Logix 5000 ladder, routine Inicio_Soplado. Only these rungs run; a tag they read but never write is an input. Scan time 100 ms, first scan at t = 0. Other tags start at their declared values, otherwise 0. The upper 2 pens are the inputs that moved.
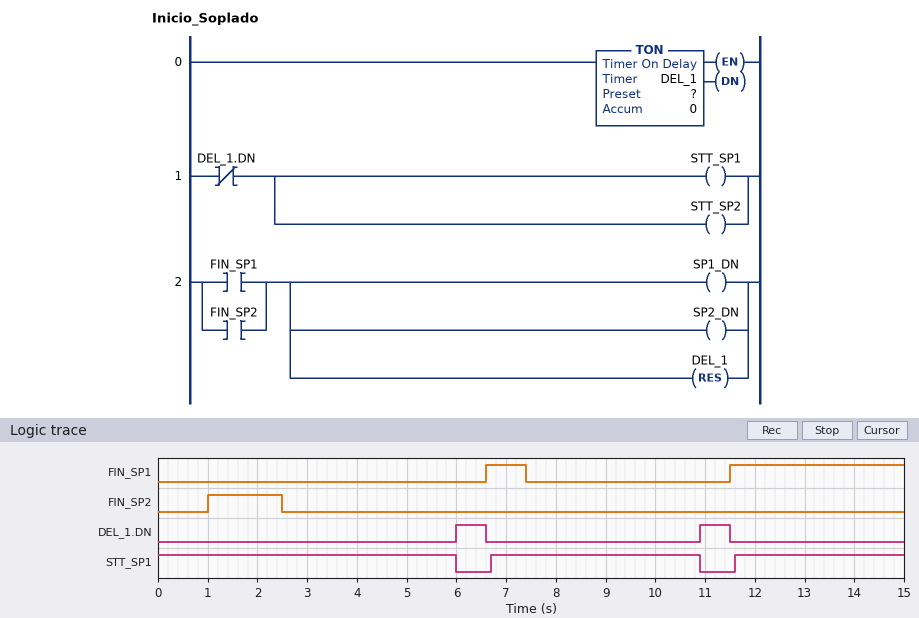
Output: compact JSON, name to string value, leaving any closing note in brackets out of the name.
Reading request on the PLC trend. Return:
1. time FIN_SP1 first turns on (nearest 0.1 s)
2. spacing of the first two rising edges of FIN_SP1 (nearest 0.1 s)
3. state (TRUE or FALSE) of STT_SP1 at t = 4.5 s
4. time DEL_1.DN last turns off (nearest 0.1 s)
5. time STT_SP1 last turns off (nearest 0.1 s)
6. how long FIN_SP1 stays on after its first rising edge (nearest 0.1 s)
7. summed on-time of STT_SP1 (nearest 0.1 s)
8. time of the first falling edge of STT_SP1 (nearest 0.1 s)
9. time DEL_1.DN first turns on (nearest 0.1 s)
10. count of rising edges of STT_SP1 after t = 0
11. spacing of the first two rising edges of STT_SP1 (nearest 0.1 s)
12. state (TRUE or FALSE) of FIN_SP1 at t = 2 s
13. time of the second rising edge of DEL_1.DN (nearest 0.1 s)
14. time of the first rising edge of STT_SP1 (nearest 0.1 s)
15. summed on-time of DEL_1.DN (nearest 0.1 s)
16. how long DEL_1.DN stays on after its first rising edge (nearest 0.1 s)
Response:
{"time FIN_SP1 first turns on": "6.6 s", "spacing of the first two rising edges of FIN_SP1": "4.9 s", "state (TRUE or FALSE) of STT_SP1 at t = 4.5 s": "TRUE", "time DEL_1.DN last turns off": "11.5 s", "time STT_SP1 last turns off": "10.9 s", "how long FIN_SP1 stays on after its first rising edge": "0.8 s", "summed on-time of STT_SP1": "13.6 s", "time of the first falling edge of STT_SP1": "6.0 s", "time DEL_1.DN first turns on": "6.0 s", "count of rising edges of STT_SP1 after t = 0": "2", "spacing of the first two rising edges of STT_SP1": "4.9 s", "state (TRUE or FALSE) of FIN_SP1 at t = 2 s": "FALSE", "time of the second rising edge of DEL_1.DN": "10.9 s", "time of the first rising edge of STT_SP1": "6.7 s", "summed on-time of DEL_1.DN": "1.2 s", "how long DEL_1.DN stays on after its first rising edge": "0.6 s"}
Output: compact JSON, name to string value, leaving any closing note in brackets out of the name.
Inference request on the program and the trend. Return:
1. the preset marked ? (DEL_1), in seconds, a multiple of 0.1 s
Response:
{"the preset marked ? (DEL_1), in seconds, a multiple of 0.1 s": "3.5 s"}
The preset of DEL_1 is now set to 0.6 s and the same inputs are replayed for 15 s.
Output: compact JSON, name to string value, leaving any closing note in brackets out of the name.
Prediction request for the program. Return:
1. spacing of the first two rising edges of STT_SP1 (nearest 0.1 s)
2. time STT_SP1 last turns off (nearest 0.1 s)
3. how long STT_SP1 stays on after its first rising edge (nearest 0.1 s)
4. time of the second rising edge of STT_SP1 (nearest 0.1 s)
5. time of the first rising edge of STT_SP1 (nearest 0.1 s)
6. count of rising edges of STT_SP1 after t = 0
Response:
{"spacing of the first two rising edges of STT_SP1": "5.6 s", "time STT_SP1 last turns off": "8.0 s", "how long STT_SP1 stays on after its first rising edge": "2.0 s", "time of the second rising edge of STT_SP1": "6.7 s", "time of the first rising edge of STT_SP1": "1.1 s", "count of rising edges of STT_SP1 after t = 0": "3"}
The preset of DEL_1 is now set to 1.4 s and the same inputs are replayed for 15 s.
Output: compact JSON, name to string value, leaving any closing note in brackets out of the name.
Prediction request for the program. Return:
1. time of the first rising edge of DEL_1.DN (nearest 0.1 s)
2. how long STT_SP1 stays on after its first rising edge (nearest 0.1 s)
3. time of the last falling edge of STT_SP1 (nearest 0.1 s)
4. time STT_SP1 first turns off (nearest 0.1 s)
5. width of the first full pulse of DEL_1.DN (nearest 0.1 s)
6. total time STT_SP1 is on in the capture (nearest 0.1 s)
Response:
{"time of the first rising edge of DEL_1.DN": "3.9 s", "how long STT_SP1 stays on after its first rising edge": "2.1 s", "time of the last falling edge of STT_SP1": "8.8 s", "time STT_SP1 first turns off": "3.9 s", "width of the first full pulse of DEL_1.DN": "2.7 s", "total time STT_SP1 is on in the capture": "9.4 s"}
